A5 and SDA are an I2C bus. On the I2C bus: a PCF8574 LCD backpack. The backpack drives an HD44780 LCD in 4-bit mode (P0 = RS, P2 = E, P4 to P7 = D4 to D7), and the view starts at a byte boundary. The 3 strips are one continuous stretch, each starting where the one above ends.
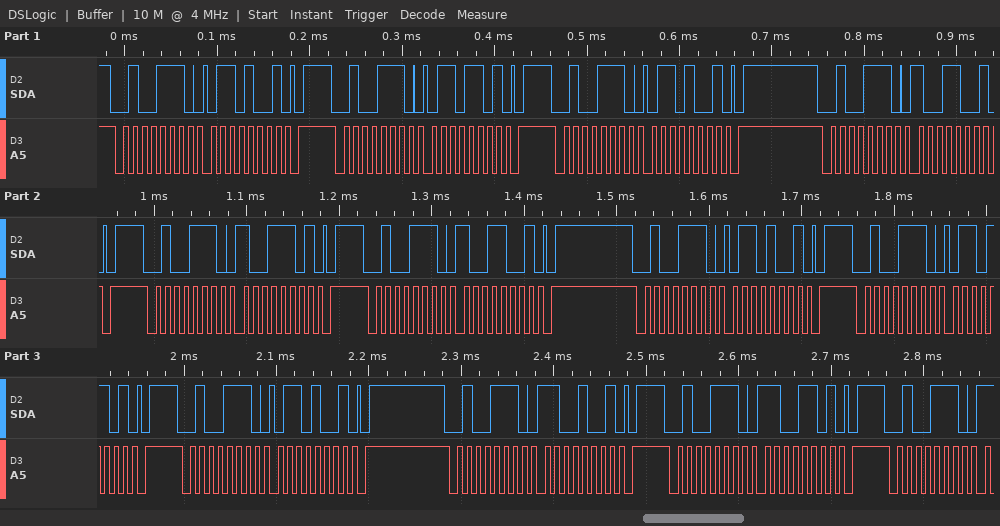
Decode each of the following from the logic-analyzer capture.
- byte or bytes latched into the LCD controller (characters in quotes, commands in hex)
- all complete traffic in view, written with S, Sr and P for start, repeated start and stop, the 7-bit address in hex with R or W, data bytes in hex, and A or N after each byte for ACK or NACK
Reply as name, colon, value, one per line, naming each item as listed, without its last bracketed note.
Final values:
byte or bytes latched into the LCD controller: 'i'
all complete traffic in view, written with S, Sr and P for start, repeated start and stop, the 7-bit address in hex with R or W, data bytes in hex, and A or N after each byte for ACK or NACK: S 27W A 69 A P S 27W A 6D A P S 27W A 69 A P S 27W A 99 A P S 27W A 9D A P S 27W A 99 A P S 27W A 69 A P S 27W A 6D A P S 27W A 69 A P S 27W A C9 A P S 27W A CD A P S 27W A
